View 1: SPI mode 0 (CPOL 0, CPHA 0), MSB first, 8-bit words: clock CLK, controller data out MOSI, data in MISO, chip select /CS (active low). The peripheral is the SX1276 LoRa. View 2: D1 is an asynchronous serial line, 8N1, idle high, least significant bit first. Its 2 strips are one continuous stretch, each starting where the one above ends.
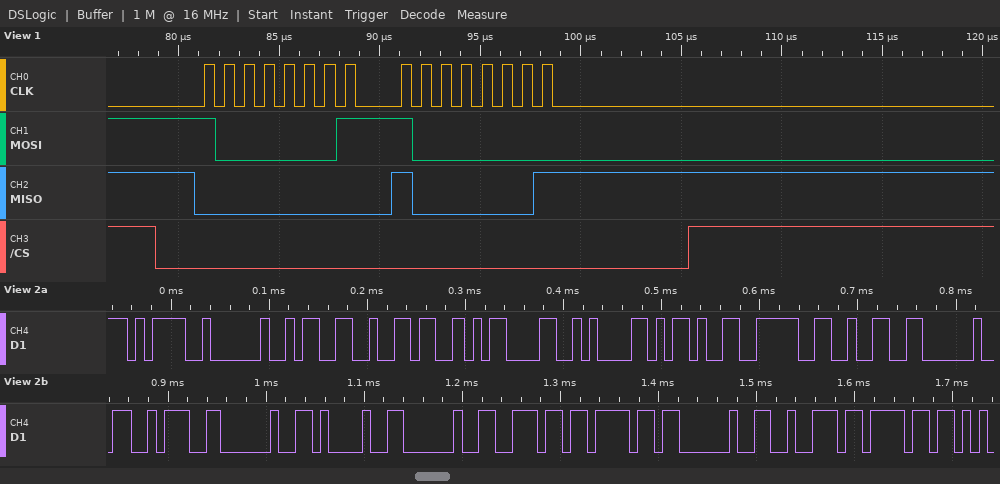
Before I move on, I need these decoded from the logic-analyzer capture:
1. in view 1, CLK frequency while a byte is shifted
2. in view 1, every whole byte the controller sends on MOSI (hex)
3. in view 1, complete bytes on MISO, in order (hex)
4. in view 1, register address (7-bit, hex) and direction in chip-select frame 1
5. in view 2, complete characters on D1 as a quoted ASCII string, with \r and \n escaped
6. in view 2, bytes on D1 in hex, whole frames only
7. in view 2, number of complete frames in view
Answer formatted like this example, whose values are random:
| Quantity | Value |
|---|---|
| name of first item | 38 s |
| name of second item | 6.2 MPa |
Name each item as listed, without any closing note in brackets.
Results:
| Quantity | Value |
|---|---|
| in view 1, CLK frequency while a byte is shifted | 1 MHz |
| in view 1, every whole byte the controller sends on MOSI | 81 80 |
| in view 1, complete bytes on MISO, in order | 00 81 |
| in view 1, register address (7-bit, hex) and direction in chip-select frame 1 | 0x01 write |
| in view 2, complete characters on D1 as a quoted ASCII string, with \r and \n escaped | "= 36\r\n->2 : ! no ro" |
| in view 2, bytes on D1 in hex, whole frames only | 3D 20 33 36 0D 0A 2D 3E 32 20 3A 20 21 20 6E 6F 20 72 6F |
| in view 2, number of complete frames in view | 19 |
